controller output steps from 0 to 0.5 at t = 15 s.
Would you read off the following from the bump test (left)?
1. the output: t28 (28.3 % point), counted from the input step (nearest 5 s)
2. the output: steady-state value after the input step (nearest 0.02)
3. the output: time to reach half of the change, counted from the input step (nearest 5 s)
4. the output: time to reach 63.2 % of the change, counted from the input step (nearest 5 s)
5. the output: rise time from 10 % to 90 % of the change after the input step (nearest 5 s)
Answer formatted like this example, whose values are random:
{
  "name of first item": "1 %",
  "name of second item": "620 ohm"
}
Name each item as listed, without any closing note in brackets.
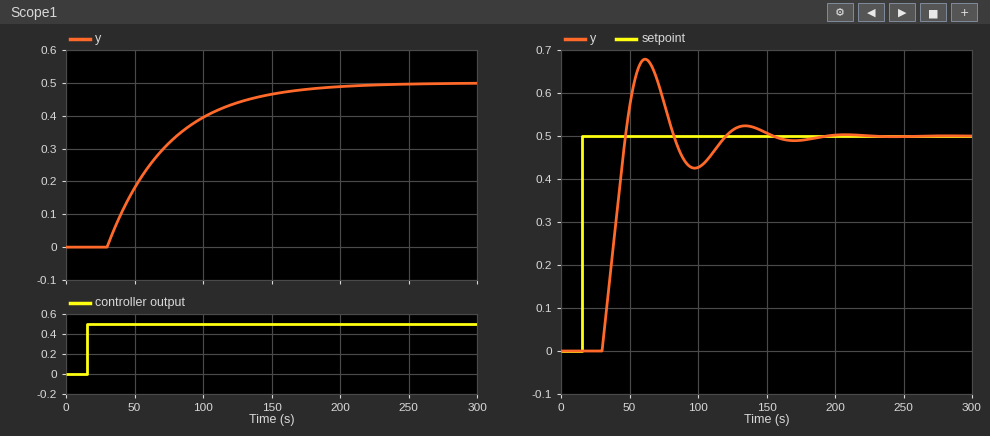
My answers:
{
  "the output: t28 (28.3 % point), counted from the input step": "30 s",
  "the output: steady-state value after the input step": "0.50",
  "the output: time to reach half of the change, counted from the input step": "45 s",
  "the output: time to reach 63.2 % of the change, counted from the input step": "60 s",
  "the output: rise time from 10 % to 90 % of the change after the input step": "100 s"
}
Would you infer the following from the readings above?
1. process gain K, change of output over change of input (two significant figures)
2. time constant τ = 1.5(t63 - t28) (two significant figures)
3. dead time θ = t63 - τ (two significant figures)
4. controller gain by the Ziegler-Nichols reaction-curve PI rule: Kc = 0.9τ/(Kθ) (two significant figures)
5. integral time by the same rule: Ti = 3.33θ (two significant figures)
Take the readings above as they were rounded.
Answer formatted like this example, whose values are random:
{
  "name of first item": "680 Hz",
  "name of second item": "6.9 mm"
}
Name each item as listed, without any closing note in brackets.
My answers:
{
  "process gain K, change of output over change of input": "1.0",
  "time constant τ = 1.5(t63 - t28)": "45 s",
  "dead time θ = t63 - τ": "15 s",
  "controller gain by the Ziegler-Nichols reaction-curve PI rule: Kc = 0.9τ/(Kθ)": "2.7",
  "integral time by the same rule: Ti = 3.33θ": "50 s"
}
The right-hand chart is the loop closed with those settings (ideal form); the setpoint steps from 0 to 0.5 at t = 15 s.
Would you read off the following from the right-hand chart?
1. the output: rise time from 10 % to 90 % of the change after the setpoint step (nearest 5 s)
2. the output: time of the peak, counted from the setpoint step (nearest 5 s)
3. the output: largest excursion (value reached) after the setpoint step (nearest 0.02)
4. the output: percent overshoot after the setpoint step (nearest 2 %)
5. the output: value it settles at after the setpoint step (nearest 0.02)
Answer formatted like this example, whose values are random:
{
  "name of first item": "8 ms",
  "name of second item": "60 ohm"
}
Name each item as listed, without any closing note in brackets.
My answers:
{
  "the output: rise time from 10 % to 90 % of the change after the setpoint step": "15 s",
  "the output: time of the peak, counted from the setpoint step": "45 s",
  "the output: largest excursion (value reached) after the setpoint step": "0.68",
  "the output: percent overshoot after the setpoint step": "36 %",
  "the output: value it settles at after the setpoint step": "0.50"
}
